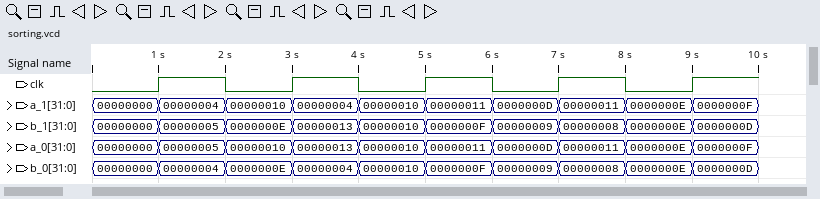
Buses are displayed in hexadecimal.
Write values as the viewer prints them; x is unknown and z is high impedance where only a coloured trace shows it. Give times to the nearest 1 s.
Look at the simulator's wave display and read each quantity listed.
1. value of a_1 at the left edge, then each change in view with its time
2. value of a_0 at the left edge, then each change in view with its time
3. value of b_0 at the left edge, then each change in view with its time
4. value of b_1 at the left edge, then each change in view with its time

00000000, 00000004 at 1 s, 00000010 at 2 s, 00000004 at 3 s, 00000010 at 4 s, 00000011 at 5 s, 0000000D at 6 s, 00000011 at 7 s, 0000000E at 8 s, 0000000F at 9 s
00000000, 00000005 at 1 s, 00000010 at 2 s, 00000013 at 3 s, 00000010 at 4 s, 00000011 at 5 s, 0000000D at 6 s, 00000011 at 7 s, 0000000E at 8 s, 0000000F at 9 s
00000000, 00000004 at 1 s, 0000000E at 2 s, 00000004 at 3 s, 00000010 at 4 s, 0000000F at 5 s, 00000009 at 6 s, 00000008 at 7 s, 0000000E at 8 s, 0000000D at 9 s
00000000, 00000005 at 1 s, 0000000E at 2 s, 00000013 at 3 s, 00000010 at 4 s, 0000000F at 5 s, 00000009 at 6 s, 00000008 at 7 s, 0000000E at 8 s, 0000000D at 9 s
